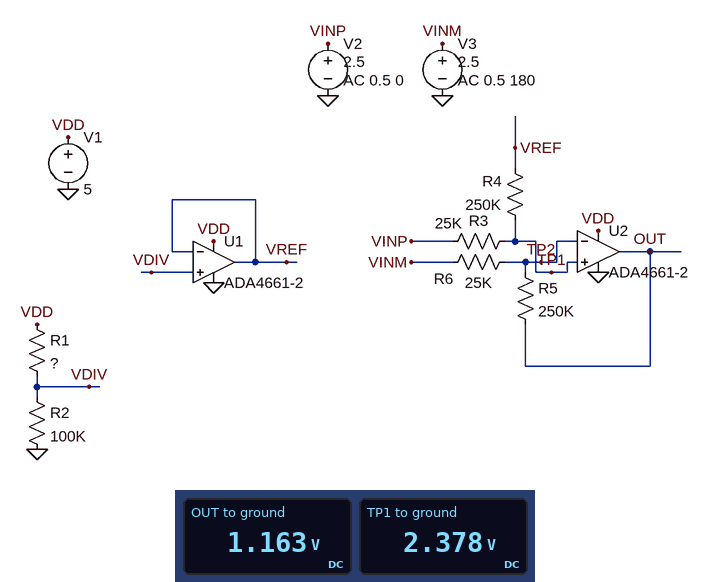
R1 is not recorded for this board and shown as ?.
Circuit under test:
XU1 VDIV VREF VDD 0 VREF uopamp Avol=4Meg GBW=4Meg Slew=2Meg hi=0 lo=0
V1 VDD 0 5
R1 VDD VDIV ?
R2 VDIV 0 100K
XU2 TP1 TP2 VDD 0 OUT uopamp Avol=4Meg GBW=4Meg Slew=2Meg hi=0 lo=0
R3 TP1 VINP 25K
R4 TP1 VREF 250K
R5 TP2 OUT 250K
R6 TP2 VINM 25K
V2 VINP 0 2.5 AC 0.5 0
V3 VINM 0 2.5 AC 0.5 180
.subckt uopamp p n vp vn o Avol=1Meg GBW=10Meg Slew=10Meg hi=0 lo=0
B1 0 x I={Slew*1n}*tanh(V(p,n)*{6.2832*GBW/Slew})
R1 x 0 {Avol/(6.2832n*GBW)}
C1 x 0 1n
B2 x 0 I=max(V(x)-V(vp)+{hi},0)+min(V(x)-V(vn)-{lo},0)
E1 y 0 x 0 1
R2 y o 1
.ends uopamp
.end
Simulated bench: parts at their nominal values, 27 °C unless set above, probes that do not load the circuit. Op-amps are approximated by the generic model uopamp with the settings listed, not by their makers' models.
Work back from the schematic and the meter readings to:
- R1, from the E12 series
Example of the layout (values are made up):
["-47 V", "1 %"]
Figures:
["330 kΩ"]
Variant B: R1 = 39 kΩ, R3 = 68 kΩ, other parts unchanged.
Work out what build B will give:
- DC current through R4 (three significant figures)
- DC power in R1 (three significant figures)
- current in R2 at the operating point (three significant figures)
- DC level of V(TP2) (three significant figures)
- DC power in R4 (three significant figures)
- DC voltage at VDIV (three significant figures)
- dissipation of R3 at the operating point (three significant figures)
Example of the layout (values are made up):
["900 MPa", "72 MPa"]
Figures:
["3.45 µA", "50.5 µW", "36.0 µA", "2.73 V", "2.98 µW", "3.60 V", "809 nW"]
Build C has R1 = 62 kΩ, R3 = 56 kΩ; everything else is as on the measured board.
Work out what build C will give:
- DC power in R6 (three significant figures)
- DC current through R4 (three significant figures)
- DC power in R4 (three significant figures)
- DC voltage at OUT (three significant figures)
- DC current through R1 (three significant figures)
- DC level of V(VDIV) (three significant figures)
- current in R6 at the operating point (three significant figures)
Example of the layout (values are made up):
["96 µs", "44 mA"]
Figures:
["461 nW", "1.92 µA", "918 nW", "3.68 V", "30.9 µA", "3.09 V", "4.29 µA"]
